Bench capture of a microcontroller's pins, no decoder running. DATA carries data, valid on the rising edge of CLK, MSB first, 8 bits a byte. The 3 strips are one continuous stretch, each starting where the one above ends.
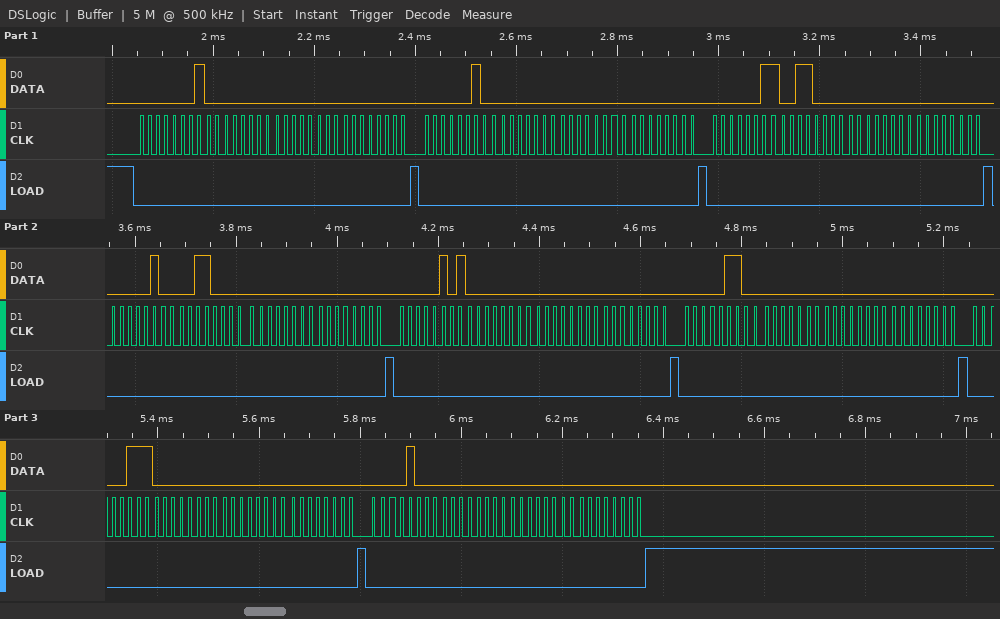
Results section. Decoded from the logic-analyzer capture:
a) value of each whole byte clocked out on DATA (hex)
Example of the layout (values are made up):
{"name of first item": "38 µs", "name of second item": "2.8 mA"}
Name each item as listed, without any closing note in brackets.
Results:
{"value of each whole byte clocked out on DATA": "0x01 0x00 0x00 0x00 0x02 0x00 0x00 0x00 0x03 0x30 0x00 0x00 0x04 0x30 0x00 0x00 0x05 0x00 0x00 0x00 0x06 0x00 0x00 0x00 0x07 0x00 0x00 0x00 0x08 0x00 0x00 0x00"}
